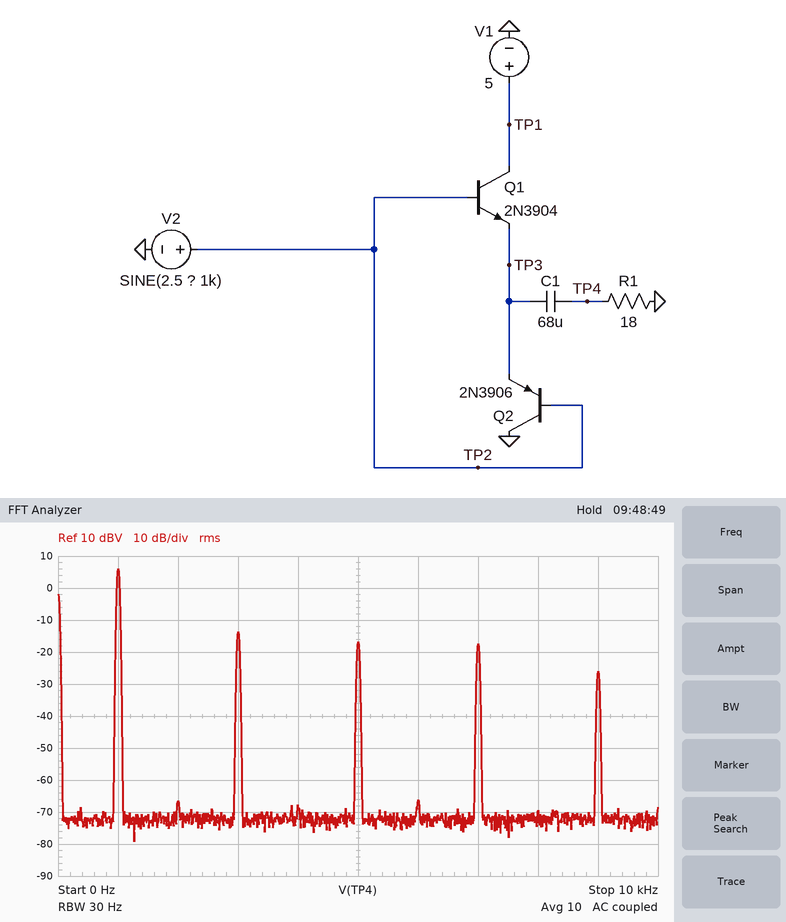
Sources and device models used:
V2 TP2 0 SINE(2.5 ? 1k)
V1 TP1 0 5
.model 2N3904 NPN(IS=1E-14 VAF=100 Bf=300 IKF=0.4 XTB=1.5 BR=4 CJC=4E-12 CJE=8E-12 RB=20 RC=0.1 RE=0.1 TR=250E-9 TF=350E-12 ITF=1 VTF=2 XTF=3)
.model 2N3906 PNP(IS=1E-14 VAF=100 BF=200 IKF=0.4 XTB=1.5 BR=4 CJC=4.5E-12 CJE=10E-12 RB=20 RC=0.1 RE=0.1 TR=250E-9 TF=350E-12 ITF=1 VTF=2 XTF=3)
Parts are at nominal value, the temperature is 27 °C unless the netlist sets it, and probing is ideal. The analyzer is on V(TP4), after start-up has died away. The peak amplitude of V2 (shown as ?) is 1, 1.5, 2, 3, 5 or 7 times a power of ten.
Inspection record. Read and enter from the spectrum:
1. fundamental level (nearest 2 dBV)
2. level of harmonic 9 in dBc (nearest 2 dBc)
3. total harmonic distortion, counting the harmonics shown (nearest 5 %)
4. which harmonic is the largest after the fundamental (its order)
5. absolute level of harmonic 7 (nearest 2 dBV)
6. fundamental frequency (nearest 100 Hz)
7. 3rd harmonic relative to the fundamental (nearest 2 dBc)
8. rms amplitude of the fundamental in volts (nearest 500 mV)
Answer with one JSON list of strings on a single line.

["6 dBV", "-32 dBc", "15 %", "3", "-18 dBV", "1.0 kHz", "-20 dBc", "2.0 V"]
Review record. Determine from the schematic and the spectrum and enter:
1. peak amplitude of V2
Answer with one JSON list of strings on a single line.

["5 V"]
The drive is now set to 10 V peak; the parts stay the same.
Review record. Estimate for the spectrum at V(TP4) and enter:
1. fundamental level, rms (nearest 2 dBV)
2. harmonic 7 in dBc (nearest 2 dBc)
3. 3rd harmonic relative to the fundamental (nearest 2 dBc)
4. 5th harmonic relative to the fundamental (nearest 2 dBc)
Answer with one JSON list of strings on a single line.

["6 dBV", "-32 dBc", "-12 dBc", "-20 dBc"]
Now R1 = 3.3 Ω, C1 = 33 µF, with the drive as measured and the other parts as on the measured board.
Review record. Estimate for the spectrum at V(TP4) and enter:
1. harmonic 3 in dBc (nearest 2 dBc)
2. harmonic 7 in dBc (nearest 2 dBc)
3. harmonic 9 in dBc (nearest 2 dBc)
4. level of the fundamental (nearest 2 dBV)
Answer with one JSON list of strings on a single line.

["-10 dBc", "-38 dBc", "-28 dBc", "2 dBV"]
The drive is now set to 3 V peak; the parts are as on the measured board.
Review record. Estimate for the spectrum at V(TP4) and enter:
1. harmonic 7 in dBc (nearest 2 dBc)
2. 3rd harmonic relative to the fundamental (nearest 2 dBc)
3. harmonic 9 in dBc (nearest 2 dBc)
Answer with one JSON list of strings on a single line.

["-30 dBc", "-18 dBc", "-36 dBc"]
